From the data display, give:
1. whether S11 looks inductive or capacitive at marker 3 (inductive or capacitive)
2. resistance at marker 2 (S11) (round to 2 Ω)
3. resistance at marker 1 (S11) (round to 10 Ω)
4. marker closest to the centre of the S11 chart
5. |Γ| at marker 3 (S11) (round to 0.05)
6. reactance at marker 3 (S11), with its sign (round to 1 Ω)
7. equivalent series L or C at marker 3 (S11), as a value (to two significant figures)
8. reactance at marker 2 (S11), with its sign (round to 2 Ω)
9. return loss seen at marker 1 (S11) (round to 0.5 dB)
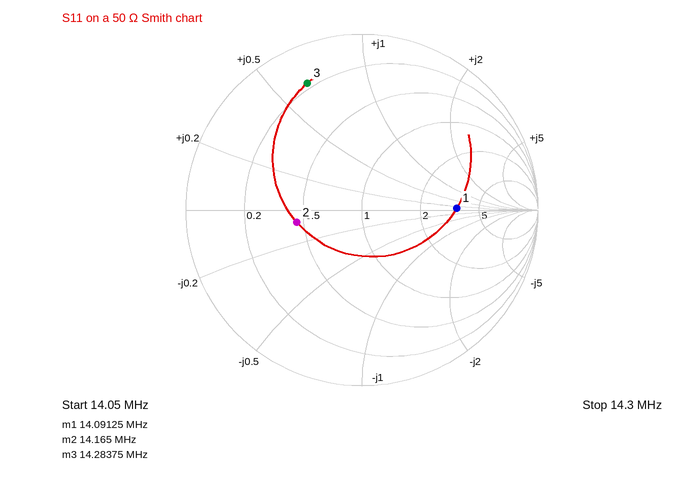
inductive
22 Ω
170 Ω
marker 2
0.80
+32 Ω
360 nH
-4 Ω
5.5 dB
